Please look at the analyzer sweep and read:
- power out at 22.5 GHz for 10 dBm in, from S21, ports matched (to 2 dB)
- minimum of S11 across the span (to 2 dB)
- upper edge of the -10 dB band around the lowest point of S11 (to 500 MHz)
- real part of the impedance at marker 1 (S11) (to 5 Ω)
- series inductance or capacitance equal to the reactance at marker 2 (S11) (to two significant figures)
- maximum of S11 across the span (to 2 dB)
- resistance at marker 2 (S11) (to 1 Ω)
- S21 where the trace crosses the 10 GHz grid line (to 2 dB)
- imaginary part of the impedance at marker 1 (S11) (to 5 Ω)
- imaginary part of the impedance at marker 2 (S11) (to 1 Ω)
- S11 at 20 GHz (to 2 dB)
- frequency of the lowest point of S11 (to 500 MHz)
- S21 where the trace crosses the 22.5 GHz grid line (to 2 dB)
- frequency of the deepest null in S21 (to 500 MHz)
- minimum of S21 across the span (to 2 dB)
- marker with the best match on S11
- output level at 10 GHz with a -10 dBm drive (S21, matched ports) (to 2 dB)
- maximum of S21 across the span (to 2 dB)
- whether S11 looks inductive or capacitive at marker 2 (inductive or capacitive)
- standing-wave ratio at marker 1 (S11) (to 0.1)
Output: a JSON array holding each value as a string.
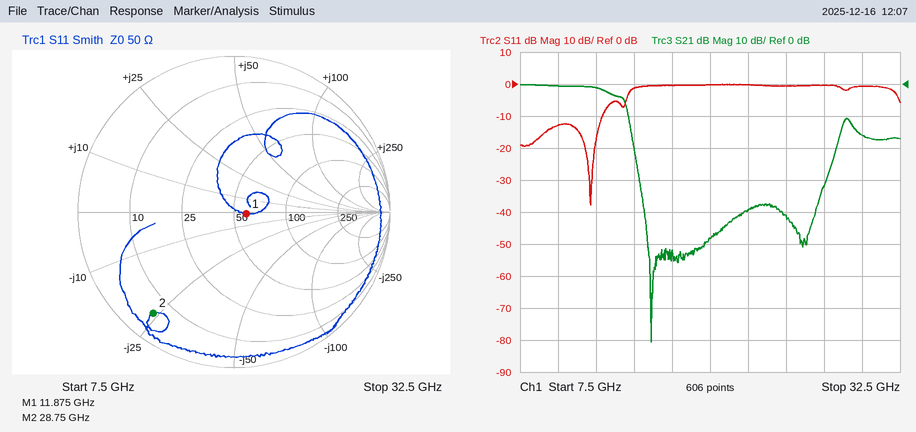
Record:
["-30 dBm", "-38 dB", "13.0 GHz", "60 Ω", "230 fF", "0 dB", "6 Ω", "0 dB", "0 Ω", "-24 Ω", "0 dB", "12.0 GHz", "-40 dB", "16.0 GHz", "-80 dB", "marker 1", "-10 dBm", "0 dB", "capacitive", "1.2"]
